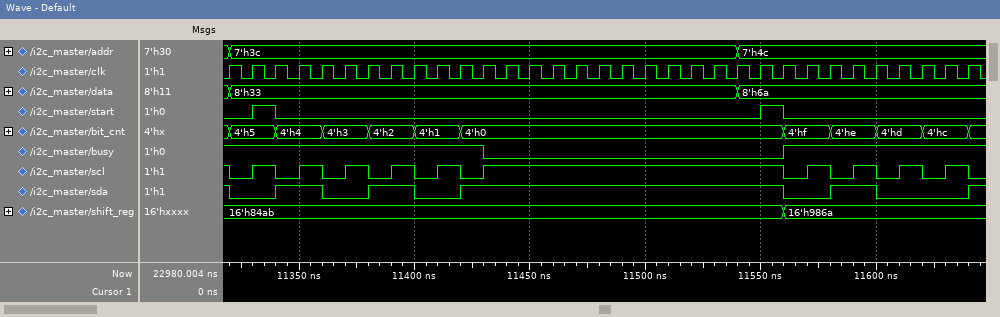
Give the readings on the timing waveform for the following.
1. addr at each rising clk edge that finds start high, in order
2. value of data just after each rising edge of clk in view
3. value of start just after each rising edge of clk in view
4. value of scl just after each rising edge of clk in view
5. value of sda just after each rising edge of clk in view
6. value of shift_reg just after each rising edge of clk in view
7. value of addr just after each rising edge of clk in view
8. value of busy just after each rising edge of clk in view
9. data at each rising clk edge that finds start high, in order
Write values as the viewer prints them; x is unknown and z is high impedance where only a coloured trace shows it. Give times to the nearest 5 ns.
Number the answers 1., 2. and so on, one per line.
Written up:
1. 7'h3c, 7'h4c
2. 8'h33, 8'h33, 8'h33, 8'h33, 8'h33, 8'h33, 8'h33, 8'h33, 8'h33, 8'h33, 8'h33, 8'h33, 8'h33, 8'h33, 8'h33, 8'h33, 8'h33, 8'h33, 8'h33, 8'h33, 8'h33, 8'h33, 8'h6a, 8'h6a, 8'h6a, 8'h6a, 8'h6a, 8'h6a, 8'h6a, 8'h6a, 8'h6a, 8'h6a, 8'h6a
3. 0 1 0 0 0 0 0 0 0 0 0 0 0 0 0 0 0 0 0 0 0 0 0 1 0 0 0 0 0 0 0 0 0
4. 0 1 0 1 0 1 0 1 0 1 0 1 1 1 1 1 1 1 1 1 1 1 1 1 0 1 0 1 0 1 0 1 0
5. 0 0 1 1 0 0 1 1 0 0 1 1 1 1 1 1 1 1 1 1 1 1 1 1 0 0 1 1 0 0 0 0 1
6. 16'h84ab, 16'h84ab, 16'h84ab, 16'h84ab, 16'h84ab, 16'h84ab, 16'h84ab, 16'h84ab, 16'h84ab, 16'h84ab, 16'h84ab, 16'h84ab, 16'h84ab, 16'h84ab, 16'h84ab, 16'h84ab, 16'h84ab, 16'h84ab, 16'h84ab, 16'h84ab, 16'h84ab, 16'h84ab, 16'h84ab, 16'h84ab, 16'h986a, 16'h986a, 16'h986a, 16'h986a, 16'h986a, 16'h986a, 16'h986a, 16'h986a, 16'h986a
7. 7'h3c, 7'h3c, 7'h3c, 7'h3c, 7'h3c, 7'h3c, 7'h3c, 7'h3c, 7'h3c, 7'h3c, 7'h3c, 7'h3c, 7'h3c, 7'h3c, 7'h3c, 7'h3c, 7'h3c, 7'h3c, 7'h3c, 7'h3c, 7'h3c, 7'h3c, 7'h4c, 7'h4c, 7'h4c, 7'h4c, 7'h4c, 7'h4c, 7'h4c, 7'h4c, 7'h4c, 7'h4c, 7'h4c
8. 1 1 1 1 1 1 1 1 1 1 1 0 0 0 0 0 0 0 0 0 0 0 0 0 1 1 1 1 1 1 1 1 1
9. 8'h33, 8'h6a
